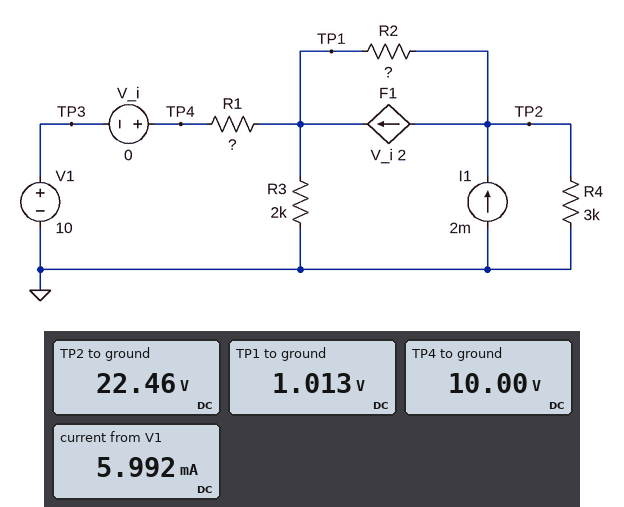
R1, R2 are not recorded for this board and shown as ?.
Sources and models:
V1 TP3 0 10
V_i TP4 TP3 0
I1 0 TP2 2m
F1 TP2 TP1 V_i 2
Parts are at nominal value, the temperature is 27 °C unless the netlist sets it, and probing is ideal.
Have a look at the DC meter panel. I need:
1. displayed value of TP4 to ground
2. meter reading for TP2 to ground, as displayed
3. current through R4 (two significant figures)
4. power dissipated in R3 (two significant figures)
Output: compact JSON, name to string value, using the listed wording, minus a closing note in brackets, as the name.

{"displayed value of TP4 to ground": "10.00 V", "meter reading for TP2 to ground, as displayed": "22.46 V", "current through R4": "7.5 mA", "power dissipated in R3": "510 µW"}
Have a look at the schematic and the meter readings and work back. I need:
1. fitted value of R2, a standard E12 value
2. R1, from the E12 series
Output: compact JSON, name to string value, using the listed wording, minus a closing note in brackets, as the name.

{"fitted value of R2, a standard E12 value": "3.3 kΩ", "R1, from the E12 series": "1.5 kΩ"}
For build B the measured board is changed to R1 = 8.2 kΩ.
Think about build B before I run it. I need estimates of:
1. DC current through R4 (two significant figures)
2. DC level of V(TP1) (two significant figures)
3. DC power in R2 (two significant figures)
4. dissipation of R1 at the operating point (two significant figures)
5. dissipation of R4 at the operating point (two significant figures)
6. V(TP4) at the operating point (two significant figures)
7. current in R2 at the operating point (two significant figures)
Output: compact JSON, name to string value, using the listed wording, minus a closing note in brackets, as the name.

{"DC current through R4": "2.4 mA", "DC level of V(TP1)": "1.4 V", "DC power in R2": "10 mW", "dissipation of R1 at the operating point": "9.1 mW", "dissipation of R4 at the operating point": "17 mW", "V(TP4) at the operating point": "10 V", "current in R2 at the operating point": "1.7 mA"}
